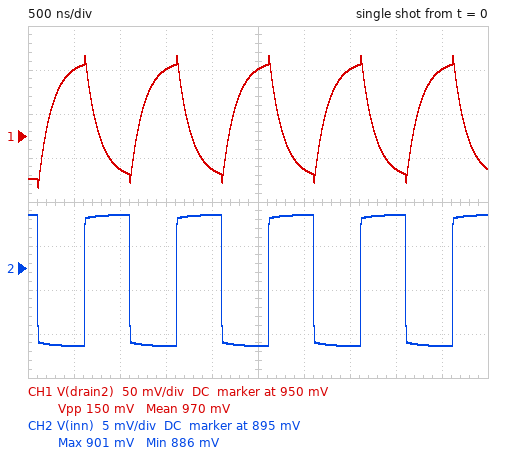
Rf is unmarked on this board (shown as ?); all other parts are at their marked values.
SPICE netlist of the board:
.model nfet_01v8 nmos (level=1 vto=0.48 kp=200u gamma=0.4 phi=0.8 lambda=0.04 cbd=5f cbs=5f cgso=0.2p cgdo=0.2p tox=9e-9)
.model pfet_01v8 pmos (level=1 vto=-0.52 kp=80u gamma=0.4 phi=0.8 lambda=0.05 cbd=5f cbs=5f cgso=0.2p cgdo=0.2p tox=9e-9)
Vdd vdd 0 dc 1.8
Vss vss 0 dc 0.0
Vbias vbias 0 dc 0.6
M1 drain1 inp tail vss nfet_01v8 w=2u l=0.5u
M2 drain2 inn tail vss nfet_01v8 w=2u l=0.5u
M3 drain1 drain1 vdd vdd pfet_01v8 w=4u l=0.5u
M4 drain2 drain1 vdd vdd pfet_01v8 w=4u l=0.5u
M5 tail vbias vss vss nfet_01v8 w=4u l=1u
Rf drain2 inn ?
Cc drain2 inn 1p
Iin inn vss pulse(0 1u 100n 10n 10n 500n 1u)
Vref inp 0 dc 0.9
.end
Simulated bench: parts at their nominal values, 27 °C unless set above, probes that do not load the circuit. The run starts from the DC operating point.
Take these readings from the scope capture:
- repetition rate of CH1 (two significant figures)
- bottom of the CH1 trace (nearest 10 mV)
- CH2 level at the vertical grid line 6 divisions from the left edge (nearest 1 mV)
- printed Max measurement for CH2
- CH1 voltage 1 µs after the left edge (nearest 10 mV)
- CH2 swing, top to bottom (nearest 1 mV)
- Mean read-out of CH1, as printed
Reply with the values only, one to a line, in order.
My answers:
1.0 MHz
890 mV
901 mV
901 mV
910 mV
15 mV
970 mV
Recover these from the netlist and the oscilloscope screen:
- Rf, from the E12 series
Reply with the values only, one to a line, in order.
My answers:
150 kΩ
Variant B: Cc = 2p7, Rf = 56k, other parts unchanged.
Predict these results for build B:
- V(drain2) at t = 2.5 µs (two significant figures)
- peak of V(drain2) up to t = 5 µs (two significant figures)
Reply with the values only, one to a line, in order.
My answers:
940 mV
950 mV
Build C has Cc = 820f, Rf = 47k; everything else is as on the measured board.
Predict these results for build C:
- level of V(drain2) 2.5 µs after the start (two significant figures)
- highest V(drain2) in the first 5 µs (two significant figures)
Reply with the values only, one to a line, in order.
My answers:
930 mV
940 mV
